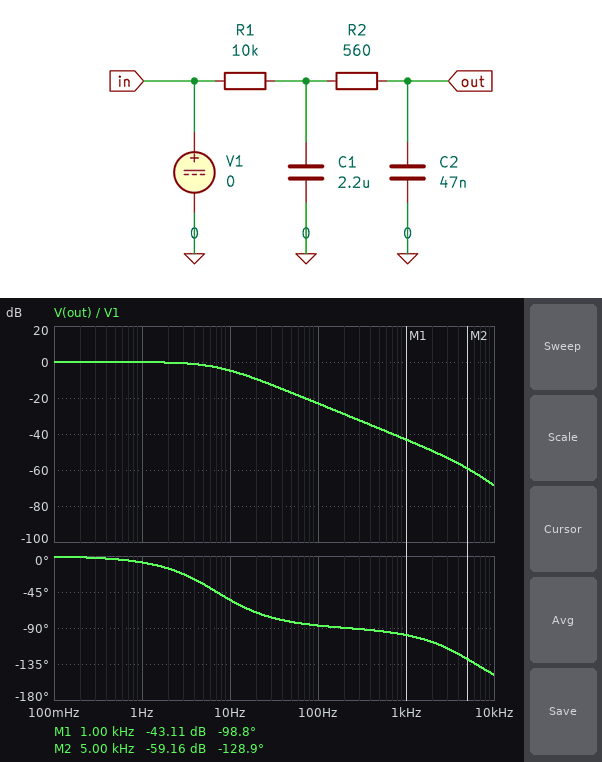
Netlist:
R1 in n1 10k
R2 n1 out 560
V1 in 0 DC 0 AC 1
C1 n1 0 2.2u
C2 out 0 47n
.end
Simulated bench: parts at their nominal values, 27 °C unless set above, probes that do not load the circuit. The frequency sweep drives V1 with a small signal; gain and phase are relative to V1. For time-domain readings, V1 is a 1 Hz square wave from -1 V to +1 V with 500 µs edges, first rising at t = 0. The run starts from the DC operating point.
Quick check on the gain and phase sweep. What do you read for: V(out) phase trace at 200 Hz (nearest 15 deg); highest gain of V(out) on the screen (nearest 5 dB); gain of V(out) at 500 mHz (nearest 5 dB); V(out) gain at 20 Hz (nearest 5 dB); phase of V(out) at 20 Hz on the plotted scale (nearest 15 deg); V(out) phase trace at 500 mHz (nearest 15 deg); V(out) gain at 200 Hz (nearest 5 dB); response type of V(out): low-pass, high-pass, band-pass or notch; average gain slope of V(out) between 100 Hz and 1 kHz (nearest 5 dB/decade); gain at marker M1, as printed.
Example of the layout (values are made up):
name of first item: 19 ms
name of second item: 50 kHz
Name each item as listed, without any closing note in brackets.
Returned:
V(out) phase trace at 200 Hz: -90 deg
highest gain of V(out) on the screen: 0 dB
gain of V(out) at 500 mHz: 0 dB
V(out) gain at 20 Hz: -10 dB
phase of V(out) at 20 Hz on the plotted scale: -75 deg
V(out) phase trace at 500 mHz: 0 deg
V(out) gain at 200 Hz: -30 dB
response type of V(out): low-pass, high-pass, band-pass or notch: low-pass
average gain slope of V(out) between 100 Hz and 1 kHz: -20 dB/decade
gain at marker M1, as printed: -43.11 dB
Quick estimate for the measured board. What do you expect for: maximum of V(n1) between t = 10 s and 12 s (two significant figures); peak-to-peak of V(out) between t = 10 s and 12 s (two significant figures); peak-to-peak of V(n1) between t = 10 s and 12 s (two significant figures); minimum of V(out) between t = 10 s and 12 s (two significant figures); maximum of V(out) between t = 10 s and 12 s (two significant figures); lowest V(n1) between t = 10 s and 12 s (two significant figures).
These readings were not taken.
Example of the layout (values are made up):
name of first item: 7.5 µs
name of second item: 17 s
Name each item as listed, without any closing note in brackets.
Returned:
maximum of V(n1) between t = 10 s and 12 s: 1.0 V
peak-to-peak of V(out) between t = 10 s and 12 s: 2.0 V
peak-to-peak of V(n1) between t = 10 s and 12 s: 2.0 V
minimum of V(out) between t = 10 s and 12 s: -1.0 V
maximum of V(out) between t = 10 s and 12 s: 1.0 V
lowest V(n1) between t = 10 s and 12 s: -1.0 V
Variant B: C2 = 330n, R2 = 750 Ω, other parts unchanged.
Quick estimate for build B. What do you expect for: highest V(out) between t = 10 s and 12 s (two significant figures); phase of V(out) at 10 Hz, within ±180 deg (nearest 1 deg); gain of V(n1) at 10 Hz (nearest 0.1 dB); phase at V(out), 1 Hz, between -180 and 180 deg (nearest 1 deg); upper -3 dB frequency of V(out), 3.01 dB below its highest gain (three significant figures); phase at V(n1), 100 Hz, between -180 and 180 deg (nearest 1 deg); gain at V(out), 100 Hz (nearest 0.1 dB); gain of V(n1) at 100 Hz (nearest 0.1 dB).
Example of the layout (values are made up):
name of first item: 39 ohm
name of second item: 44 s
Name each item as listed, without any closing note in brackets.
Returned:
highest V(out) between t = 10 s and 12 s: 1.0 V
phase of V(out) at 10 Hz, within ±180 deg: -59 deg
gain of V(n1) at 10 Hz: -5.5 dB
phase at V(out), 1 Hz, between -180 and 180 deg: -9 deg
upper -3 dB frequency of V(out), 3.01 dB below its highest gain: 6.28 Hz
phase at V(n1), 100 Hz, between -180 and 180 deg: -85 deg
gain at V(out), 100 Hz: -24.1 dB
gain of V(n1) at 100 Hz: -24.0 dB
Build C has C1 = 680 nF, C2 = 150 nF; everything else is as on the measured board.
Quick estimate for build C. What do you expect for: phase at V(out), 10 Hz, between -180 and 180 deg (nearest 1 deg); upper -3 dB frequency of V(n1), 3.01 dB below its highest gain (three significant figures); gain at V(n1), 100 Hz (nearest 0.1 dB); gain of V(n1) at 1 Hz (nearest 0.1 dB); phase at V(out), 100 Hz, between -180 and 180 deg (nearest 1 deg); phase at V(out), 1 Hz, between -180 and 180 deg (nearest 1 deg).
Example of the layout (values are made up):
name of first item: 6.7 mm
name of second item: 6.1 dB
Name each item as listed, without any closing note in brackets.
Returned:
phase at V(out), 10 Hz, between -180 and 180 deg: -28 deg
upper -3 dB frequency of V(n1), 3.01 dB below its highest gain: 19.1 Hz
gain at V(n1), 100 Hz: -14.5 dB
gain of V(n1) at 1 Hz: 0 dB
phase at V(out), 100 Hz, between -180 and 180 deg: -82 deg
phase at V(out), 1 Hz, between -180 and 180 deg: -3 deg
